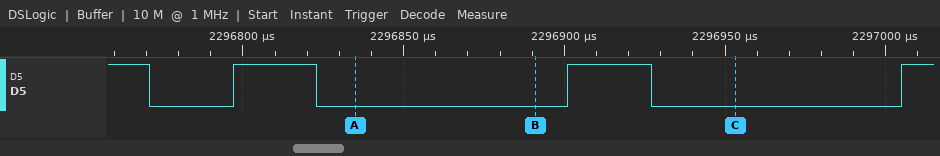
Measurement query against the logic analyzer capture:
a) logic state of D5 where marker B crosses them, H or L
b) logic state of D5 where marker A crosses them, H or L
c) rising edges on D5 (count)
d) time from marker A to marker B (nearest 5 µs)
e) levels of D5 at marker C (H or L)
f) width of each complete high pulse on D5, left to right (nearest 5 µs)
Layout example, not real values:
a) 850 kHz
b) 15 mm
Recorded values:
a) D5=L
b) D5=L
c) 3
d) 55 µs
e) D5=L
f) 25 µs, 25 µs
